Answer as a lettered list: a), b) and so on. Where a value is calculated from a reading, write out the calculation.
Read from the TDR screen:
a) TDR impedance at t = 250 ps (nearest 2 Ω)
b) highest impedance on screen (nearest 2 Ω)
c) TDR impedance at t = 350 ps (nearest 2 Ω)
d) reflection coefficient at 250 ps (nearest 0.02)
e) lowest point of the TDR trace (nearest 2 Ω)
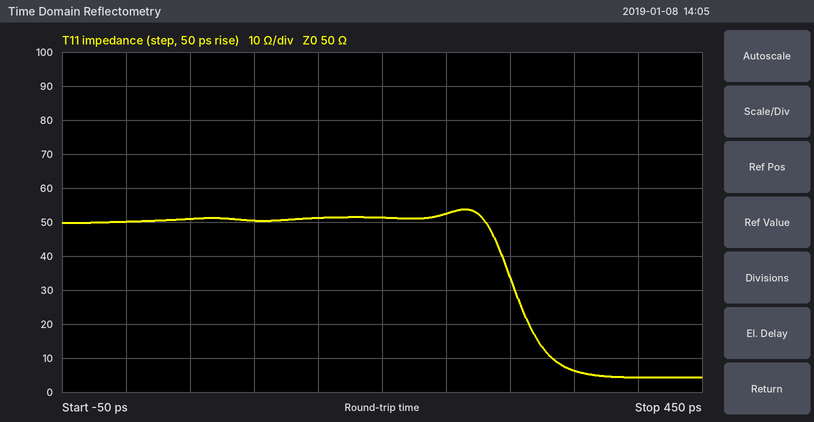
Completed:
a) 52 Ω
b) 54 Ω
c) 6 Ω
d) (52 − 50)/(52 + 50) ≈ +0.02
e) 4 Ω
